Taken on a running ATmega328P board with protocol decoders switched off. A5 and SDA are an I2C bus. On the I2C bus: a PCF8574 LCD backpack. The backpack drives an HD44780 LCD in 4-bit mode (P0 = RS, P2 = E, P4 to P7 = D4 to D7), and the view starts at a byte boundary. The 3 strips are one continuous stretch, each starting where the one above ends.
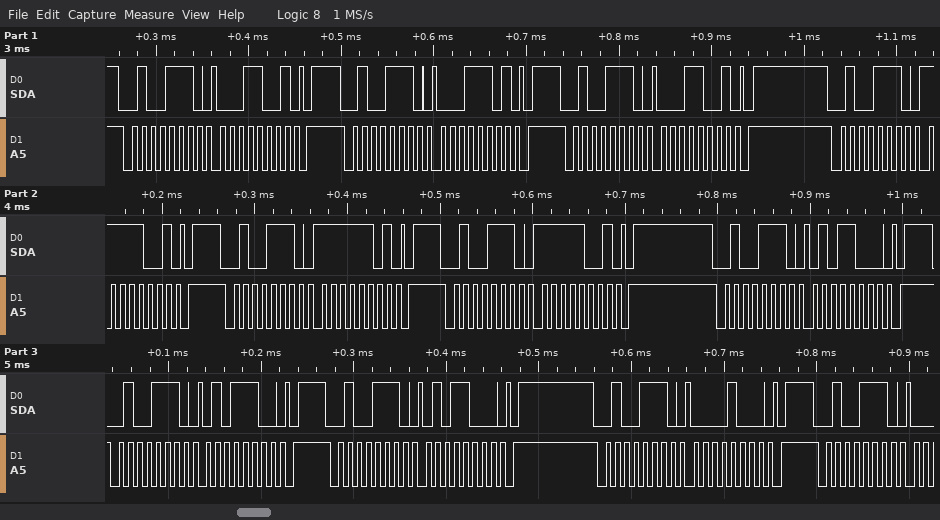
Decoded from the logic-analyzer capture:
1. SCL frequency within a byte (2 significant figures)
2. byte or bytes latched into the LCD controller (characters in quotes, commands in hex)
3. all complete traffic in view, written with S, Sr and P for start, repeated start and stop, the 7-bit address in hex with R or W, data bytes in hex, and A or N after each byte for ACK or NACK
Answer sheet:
100 kHz
data 0x1F
S 27W A 19 A P S 27W A 1D A P S 27W A 19 A P S 27W A F9 A P S 27W A FD A P S 27W A F9 A P S 27W A 58 A P S 27W A 5C A P S 27W A 58 A P S 27W A 08 A P S 27W A
